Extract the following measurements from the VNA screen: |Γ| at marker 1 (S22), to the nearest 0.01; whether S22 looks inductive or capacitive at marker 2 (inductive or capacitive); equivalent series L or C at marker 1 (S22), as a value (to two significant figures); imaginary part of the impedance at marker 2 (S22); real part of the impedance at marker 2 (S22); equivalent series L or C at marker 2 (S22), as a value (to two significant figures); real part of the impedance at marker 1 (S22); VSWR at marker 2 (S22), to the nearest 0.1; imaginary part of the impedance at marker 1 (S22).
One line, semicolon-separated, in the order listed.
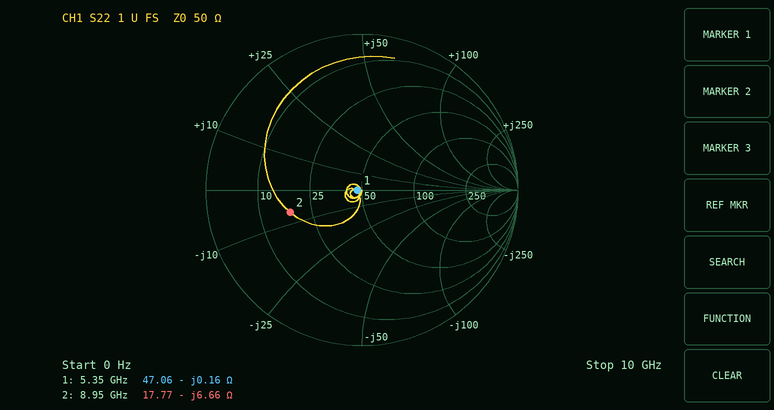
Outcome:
0.03; capacitive; 190 pF; -6.66 Ω; 17.77 Ω; 2.7 pF; 47.06 Ω; 2.9; -0.16 Ω
